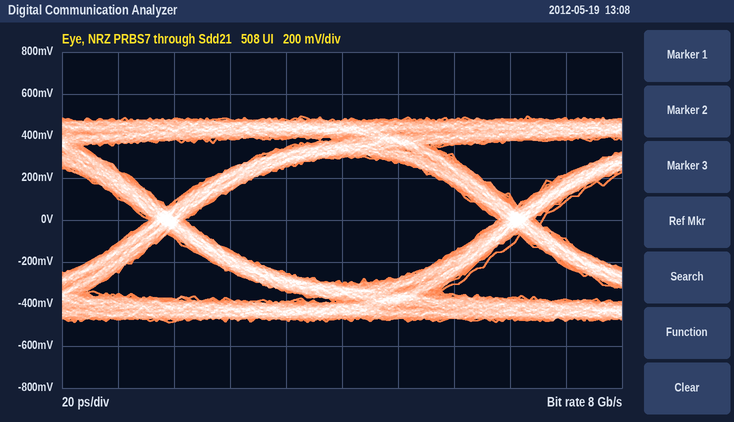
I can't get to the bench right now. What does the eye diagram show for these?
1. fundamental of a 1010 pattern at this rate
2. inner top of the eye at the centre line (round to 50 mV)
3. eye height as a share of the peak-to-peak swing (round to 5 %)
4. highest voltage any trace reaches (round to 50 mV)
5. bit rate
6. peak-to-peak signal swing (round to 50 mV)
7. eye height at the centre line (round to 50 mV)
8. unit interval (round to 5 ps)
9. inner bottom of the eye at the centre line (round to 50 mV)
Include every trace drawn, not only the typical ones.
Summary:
4 GHz
300 mV
60 %
500 mV
8 Gb/s
1.00 V
600 mV
125 ps
-300 mV
